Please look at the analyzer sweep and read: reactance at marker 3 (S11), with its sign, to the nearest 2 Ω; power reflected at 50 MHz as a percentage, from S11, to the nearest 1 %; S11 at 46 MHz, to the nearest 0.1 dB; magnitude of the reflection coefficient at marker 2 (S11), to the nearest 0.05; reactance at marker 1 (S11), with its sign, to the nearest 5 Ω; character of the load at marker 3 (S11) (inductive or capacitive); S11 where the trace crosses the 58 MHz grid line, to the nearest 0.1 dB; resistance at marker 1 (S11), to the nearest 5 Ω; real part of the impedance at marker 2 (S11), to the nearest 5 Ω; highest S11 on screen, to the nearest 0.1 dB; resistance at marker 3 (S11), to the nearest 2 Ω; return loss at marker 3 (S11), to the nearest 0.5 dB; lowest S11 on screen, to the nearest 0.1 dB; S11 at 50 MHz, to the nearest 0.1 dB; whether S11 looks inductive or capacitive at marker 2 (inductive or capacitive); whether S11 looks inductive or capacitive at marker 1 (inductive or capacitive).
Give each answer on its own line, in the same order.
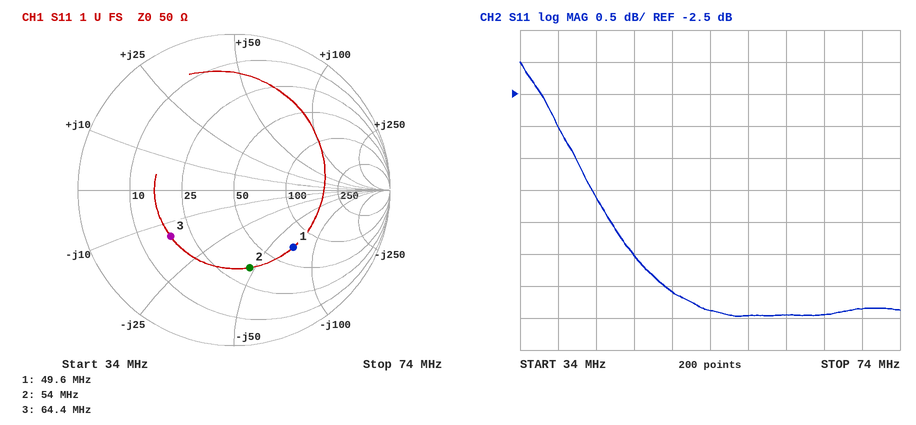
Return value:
-14 Ω
28 %
-5.0 dB
0.50
-70 Ω
capacitive
-6.0 dB
70 Ω
35 Ω
-2.0 dB
18 Ω
6.0 dB
-6.0 dB
-5.6 dB
capacitive
capacitive
